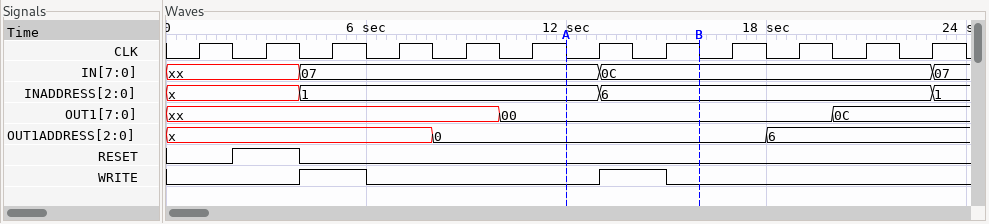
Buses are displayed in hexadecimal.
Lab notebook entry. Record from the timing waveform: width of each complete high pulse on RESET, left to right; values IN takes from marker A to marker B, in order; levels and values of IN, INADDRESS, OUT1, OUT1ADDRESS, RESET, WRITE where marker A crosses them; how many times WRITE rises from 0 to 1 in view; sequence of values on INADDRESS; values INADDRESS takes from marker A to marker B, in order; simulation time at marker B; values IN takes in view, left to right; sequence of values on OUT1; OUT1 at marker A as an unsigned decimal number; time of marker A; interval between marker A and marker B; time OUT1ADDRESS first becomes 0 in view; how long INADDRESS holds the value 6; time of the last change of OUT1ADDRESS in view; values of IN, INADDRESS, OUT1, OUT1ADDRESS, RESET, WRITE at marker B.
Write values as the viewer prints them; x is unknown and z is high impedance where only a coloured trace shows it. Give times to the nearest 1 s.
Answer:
2 s
07, 0C
IN=07, INADDRESS=1, OUT1=00, OUT1ADDRESS=0, RESET=0, WRITE=0
2
x, 1, 6, 1
1, 6
16 s
xx, 07, 0C, 07
xx, 00, 0C
0
12 s
4 s
8 s
10 s
18 s
IN=0C, INADDRESS=6, OUT1=00, OUT1ADDRESS=0, RESET=0, WRITE=0
